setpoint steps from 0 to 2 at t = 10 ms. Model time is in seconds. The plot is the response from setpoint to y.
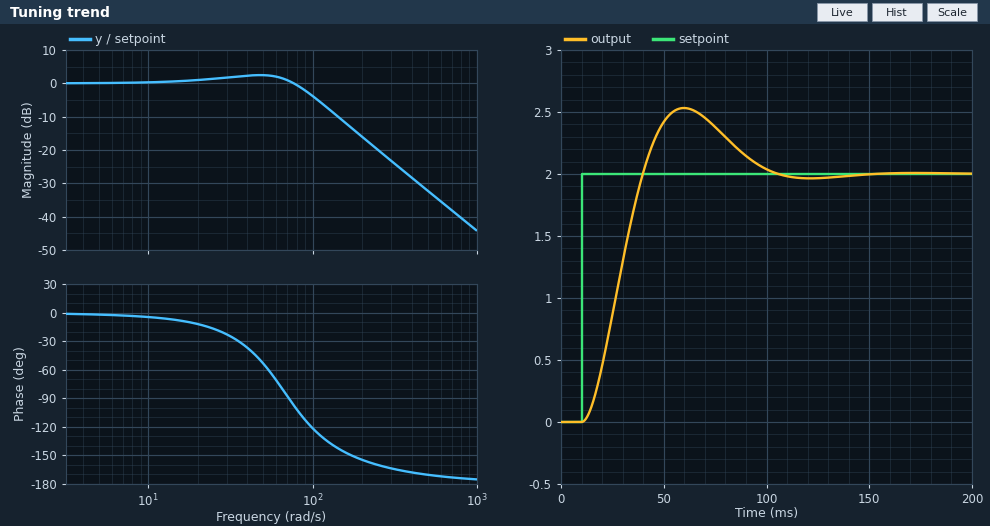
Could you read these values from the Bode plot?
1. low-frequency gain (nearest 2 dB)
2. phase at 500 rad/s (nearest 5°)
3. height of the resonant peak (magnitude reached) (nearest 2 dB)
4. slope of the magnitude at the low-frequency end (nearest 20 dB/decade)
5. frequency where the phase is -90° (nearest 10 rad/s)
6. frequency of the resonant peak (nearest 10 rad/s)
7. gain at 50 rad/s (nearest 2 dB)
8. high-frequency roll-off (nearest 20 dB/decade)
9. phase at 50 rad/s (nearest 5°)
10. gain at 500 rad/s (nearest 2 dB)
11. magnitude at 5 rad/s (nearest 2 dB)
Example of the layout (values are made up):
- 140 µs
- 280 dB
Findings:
- 0 dB
- -170°
- 2 dB
- 0 dB/decade
- 70 rad/s
- 50 rad/s
- 2 dB
- -40 dB/decade
- -55°
- -32 dB
- 0 dB
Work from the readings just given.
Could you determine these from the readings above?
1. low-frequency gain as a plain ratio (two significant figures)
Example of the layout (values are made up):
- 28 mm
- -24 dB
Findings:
- 1.0
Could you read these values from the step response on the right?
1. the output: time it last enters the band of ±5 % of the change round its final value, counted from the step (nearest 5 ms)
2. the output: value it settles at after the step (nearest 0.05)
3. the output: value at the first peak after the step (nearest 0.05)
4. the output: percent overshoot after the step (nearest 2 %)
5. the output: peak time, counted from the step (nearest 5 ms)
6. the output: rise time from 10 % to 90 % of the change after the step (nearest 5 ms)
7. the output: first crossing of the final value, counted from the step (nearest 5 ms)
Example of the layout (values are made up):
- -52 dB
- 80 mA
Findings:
- 85 ms
- 2.00
- 2.55
- 26 %
- 50 ms
- 20 ms
- 30 ms
